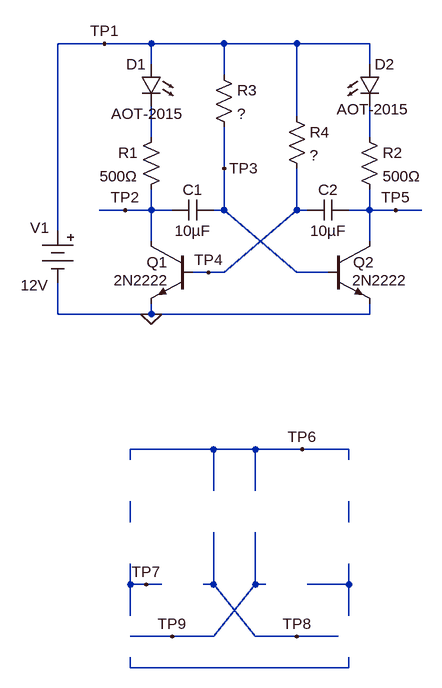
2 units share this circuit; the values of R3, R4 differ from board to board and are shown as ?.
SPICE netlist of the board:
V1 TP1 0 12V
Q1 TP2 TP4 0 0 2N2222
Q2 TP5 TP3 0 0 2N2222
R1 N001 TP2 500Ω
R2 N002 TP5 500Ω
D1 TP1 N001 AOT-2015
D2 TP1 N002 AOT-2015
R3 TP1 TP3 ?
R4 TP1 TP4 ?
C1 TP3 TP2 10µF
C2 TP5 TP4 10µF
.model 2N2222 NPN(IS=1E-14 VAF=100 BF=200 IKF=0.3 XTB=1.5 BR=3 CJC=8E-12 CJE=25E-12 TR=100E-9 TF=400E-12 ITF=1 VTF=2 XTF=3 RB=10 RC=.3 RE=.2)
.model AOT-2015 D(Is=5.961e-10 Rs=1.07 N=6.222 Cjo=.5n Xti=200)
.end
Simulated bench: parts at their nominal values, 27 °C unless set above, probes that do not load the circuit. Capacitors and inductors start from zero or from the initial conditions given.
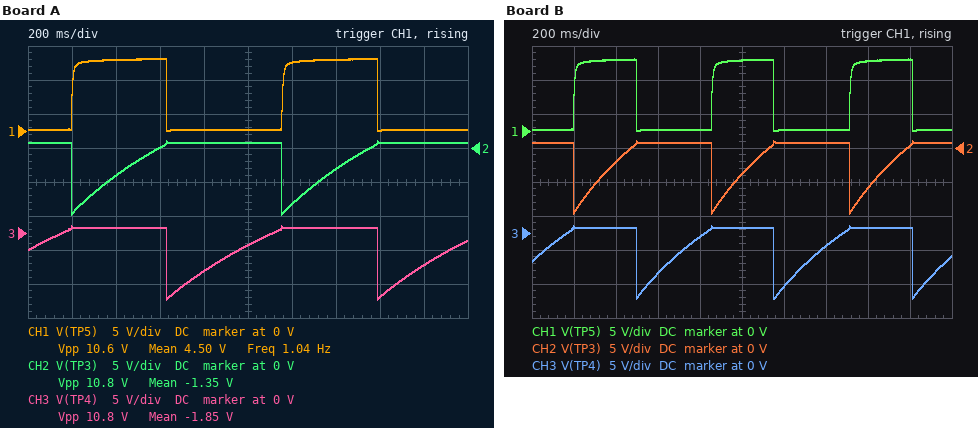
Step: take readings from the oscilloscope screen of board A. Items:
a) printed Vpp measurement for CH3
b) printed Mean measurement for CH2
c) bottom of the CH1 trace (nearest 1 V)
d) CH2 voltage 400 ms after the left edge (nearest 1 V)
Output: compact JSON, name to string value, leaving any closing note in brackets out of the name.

{"printed Vpp measurement for CH3": "10.8 V", "printed Mean measurement for CH2": "-1.35 V", "bottom of the CH1 trace": "0 V", "CH2 voltage 400 ms after the left edge": "-4 V"}
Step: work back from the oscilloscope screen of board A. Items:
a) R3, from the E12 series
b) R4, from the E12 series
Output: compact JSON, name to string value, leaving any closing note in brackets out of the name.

{"R3, from the E12 series": "68 kΩ", "R4, from the E12 series": "82 kΩ"}
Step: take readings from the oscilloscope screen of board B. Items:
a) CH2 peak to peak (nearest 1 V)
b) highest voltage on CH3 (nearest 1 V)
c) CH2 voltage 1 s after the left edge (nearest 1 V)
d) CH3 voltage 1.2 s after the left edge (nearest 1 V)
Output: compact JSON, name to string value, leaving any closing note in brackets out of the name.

{"CH2 peak to peak": "11 V", "highest voltage on CH3": "1 V", "CH2 voltage 1 s after the left edge": "-4 V", "CH3 voltage 1.2 s after the left edge": "-8 V"}
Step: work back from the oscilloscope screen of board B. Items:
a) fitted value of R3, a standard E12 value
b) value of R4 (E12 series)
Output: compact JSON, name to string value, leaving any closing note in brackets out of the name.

{"fitted value of R3, a standard E12 value": "47 kΩ", "value of R4": "56 kΩ"}
